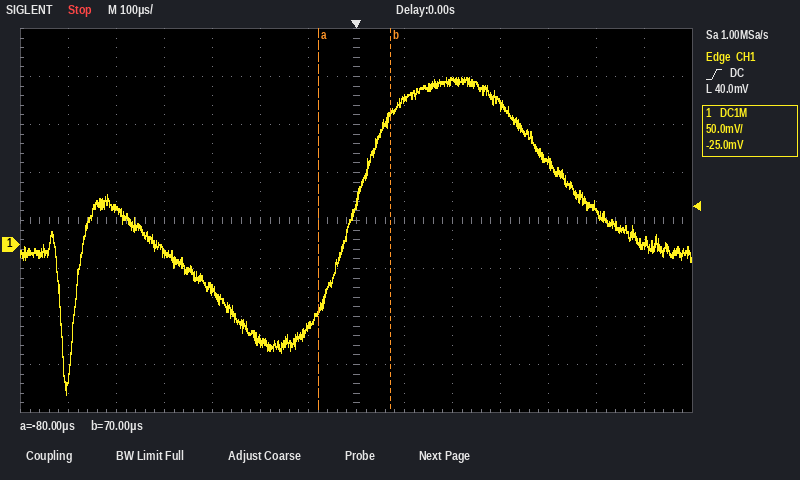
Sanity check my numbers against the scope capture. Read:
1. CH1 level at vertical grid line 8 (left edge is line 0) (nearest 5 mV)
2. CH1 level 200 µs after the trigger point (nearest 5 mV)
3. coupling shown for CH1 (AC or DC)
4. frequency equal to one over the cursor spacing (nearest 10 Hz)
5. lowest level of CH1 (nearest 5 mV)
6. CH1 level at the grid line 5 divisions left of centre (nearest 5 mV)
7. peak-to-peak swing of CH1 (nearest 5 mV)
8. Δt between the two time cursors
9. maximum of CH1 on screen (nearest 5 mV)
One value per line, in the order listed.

150 mV
170 mV
DC
6.67 kHz
-155 mV
40 mV
330 mV
150 µs
175 mV
